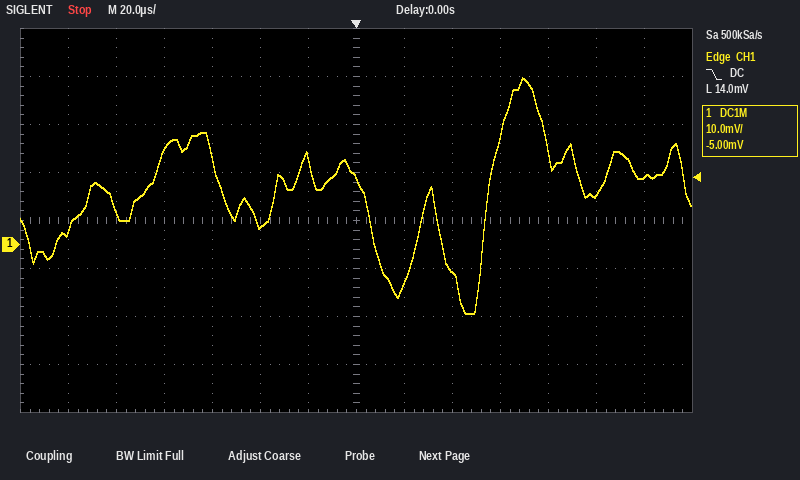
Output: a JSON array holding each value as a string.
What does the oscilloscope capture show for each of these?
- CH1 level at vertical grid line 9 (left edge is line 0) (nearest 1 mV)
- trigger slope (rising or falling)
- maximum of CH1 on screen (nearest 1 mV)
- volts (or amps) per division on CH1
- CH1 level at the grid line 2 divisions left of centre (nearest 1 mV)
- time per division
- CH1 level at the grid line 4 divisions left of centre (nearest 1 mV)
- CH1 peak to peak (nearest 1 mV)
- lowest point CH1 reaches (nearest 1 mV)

["-6 mV", "falling", "35 mV", "10 mV", "4 mV", "20 µs", "20 mV", "49 mV", "-14 mV"]
